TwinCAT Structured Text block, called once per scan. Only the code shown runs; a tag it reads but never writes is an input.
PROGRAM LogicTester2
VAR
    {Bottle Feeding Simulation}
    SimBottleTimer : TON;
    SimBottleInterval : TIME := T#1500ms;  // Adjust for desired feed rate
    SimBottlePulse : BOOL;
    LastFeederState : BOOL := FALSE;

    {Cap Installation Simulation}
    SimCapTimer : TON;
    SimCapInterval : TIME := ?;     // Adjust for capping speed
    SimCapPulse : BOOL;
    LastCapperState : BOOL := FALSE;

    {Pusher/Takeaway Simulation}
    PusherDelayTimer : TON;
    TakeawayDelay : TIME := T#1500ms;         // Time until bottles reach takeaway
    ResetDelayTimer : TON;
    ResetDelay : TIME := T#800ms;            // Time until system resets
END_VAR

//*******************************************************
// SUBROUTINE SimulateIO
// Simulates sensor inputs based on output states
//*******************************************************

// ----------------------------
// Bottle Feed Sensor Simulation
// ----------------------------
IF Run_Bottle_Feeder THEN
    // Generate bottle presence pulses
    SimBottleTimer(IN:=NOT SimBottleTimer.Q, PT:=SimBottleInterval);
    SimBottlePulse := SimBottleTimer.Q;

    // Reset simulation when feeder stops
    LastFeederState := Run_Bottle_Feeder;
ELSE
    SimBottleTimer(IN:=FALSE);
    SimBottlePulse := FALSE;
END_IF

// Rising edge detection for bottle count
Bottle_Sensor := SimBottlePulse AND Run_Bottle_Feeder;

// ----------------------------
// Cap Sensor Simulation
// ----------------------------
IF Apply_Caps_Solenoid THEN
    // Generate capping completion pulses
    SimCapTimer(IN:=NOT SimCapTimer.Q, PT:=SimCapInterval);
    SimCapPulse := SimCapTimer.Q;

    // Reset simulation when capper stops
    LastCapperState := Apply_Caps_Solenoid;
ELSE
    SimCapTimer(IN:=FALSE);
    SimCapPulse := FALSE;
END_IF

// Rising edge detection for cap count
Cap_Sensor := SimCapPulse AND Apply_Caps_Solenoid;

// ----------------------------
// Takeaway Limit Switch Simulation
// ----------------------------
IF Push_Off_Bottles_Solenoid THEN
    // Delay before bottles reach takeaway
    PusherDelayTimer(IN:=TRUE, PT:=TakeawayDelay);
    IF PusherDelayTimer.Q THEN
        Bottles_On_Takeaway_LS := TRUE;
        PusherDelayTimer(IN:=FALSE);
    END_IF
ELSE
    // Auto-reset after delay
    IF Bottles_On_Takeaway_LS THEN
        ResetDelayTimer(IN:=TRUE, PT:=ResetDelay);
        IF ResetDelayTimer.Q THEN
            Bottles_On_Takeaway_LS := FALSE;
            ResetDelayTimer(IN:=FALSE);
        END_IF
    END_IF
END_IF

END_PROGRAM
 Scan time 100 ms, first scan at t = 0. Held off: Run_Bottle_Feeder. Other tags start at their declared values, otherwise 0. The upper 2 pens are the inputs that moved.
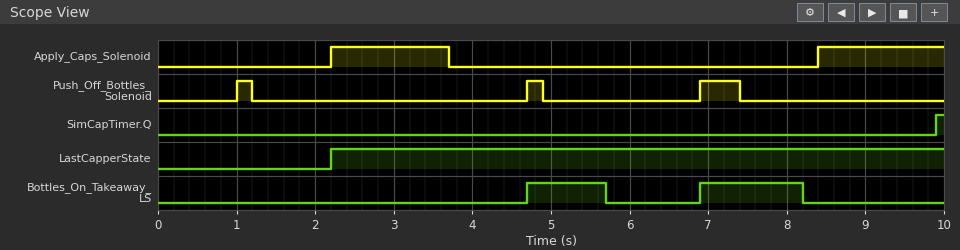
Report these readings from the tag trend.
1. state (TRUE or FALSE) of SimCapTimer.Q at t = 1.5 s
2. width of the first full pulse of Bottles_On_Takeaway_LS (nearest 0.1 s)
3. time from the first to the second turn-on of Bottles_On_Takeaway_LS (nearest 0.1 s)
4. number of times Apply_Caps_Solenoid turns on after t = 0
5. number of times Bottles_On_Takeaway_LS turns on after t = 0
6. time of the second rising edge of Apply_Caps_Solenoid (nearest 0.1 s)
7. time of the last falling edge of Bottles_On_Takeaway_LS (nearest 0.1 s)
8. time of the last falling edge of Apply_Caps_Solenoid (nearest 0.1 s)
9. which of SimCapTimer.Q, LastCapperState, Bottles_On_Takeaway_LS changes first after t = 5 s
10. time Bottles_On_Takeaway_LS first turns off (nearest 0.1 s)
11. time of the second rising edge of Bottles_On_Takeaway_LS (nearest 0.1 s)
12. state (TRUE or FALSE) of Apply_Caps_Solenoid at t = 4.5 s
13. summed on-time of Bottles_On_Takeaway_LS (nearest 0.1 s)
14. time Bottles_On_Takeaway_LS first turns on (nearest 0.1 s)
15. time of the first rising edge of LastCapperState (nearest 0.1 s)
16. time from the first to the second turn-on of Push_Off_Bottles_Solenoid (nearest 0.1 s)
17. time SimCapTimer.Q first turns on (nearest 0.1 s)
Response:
FALSE
1.0 s
2.2 s
2
2
8.4 s
8.2 s
3.7 s
Bottles_On_Takeaway_LS
5.7 s
6.9 s
FALSE
2.3 s
4.7 s
2.2 s
3.7 s
9.9 s
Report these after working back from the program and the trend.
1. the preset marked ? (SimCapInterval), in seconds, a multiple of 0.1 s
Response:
1.5 s
